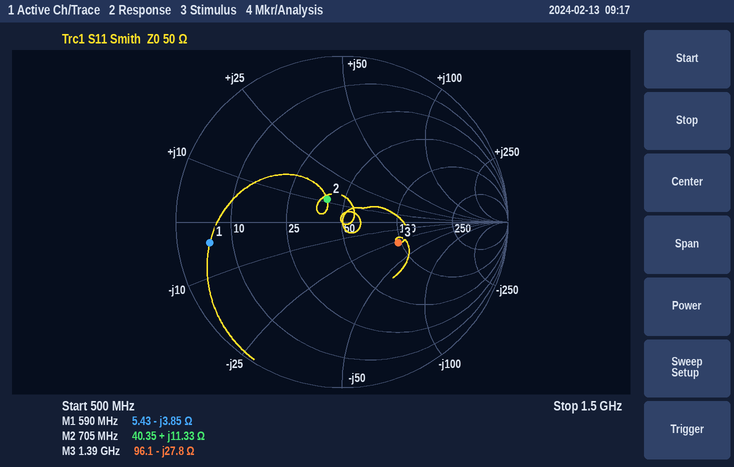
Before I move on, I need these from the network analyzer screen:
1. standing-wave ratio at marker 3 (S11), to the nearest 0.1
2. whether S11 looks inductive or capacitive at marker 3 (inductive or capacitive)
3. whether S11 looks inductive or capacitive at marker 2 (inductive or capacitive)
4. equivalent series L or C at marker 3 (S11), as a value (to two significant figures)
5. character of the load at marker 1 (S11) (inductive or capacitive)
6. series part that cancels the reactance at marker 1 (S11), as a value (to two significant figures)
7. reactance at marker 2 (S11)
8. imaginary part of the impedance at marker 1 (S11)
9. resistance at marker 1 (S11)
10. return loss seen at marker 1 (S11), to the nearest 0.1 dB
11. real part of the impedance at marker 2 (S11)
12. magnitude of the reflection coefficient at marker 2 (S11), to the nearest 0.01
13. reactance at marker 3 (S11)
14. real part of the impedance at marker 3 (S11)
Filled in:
2.1
capacitive
inductive
4.1 pF
capacitive
1.0 nH
+11.33 Ω
-3.85 Ω
5.43 Ω
1.9 dB
40.35 Ω
0.16
-27.8 Ω
96.1 Ω
